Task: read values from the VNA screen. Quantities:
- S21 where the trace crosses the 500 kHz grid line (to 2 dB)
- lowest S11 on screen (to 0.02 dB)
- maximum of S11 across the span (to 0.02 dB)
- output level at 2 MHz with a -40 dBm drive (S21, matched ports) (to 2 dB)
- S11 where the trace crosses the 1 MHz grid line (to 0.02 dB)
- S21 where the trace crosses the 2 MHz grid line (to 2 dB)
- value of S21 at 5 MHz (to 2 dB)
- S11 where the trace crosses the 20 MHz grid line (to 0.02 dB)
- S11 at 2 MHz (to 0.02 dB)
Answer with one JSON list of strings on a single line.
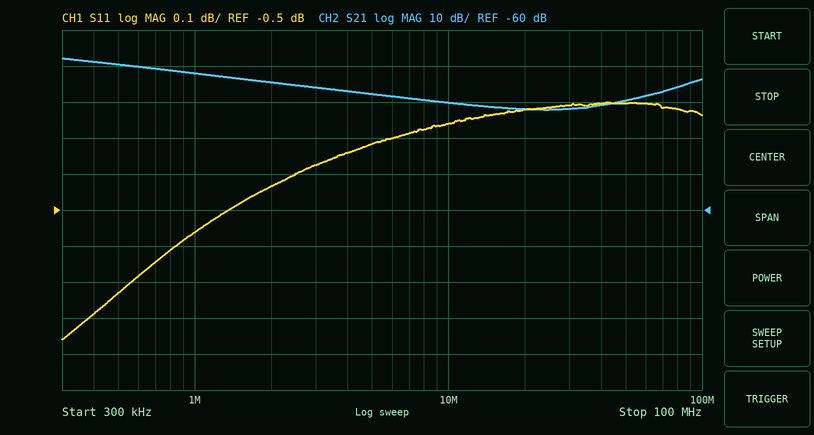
["-20 dB", "-0.86 dB", "-0.20 dB", "-64 dBm", "-0.56 dB", "-24 dB", "-28 dB", "-0.22 dB", "-0.44 dB"]
